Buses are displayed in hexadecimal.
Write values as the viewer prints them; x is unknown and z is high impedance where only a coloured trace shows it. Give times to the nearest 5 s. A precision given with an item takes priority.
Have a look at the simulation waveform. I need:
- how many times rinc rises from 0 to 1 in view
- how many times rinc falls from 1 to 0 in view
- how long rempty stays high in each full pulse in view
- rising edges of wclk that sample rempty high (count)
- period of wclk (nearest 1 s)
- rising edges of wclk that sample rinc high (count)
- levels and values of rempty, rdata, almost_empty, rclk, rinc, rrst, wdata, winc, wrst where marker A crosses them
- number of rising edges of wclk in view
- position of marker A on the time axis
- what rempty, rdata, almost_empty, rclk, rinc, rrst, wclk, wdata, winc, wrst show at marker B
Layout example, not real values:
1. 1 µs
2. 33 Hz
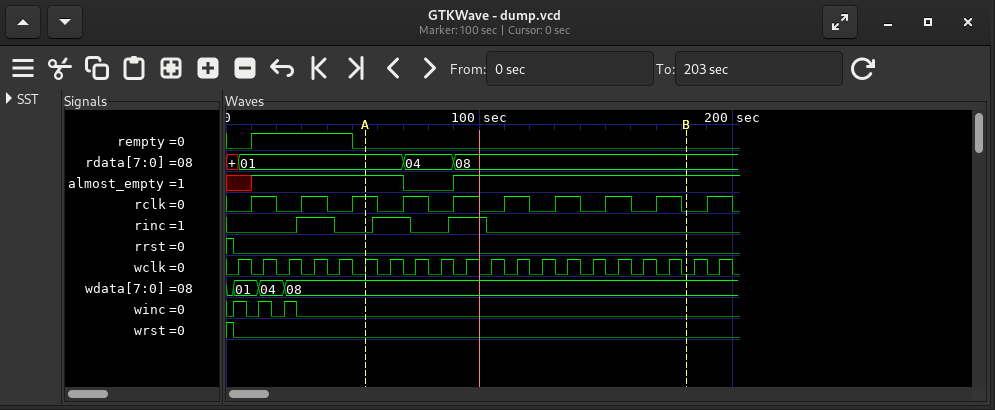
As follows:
1. 3
2. 3
3. 40 s
4. 4
5. 10 s
6. 3
7. rempty=0, rdata=01, almost_empty=1, rclk=1, rinc=0, rrst=0, wdata=08, winc=0, wrst=0
8. 20
9. 55 s
10. rempty=0, rdata=08, almost_empty=1, rclk=0, rinc=0, rrst=0, wclk=0, wdata=08, winc=0, wrst=0
